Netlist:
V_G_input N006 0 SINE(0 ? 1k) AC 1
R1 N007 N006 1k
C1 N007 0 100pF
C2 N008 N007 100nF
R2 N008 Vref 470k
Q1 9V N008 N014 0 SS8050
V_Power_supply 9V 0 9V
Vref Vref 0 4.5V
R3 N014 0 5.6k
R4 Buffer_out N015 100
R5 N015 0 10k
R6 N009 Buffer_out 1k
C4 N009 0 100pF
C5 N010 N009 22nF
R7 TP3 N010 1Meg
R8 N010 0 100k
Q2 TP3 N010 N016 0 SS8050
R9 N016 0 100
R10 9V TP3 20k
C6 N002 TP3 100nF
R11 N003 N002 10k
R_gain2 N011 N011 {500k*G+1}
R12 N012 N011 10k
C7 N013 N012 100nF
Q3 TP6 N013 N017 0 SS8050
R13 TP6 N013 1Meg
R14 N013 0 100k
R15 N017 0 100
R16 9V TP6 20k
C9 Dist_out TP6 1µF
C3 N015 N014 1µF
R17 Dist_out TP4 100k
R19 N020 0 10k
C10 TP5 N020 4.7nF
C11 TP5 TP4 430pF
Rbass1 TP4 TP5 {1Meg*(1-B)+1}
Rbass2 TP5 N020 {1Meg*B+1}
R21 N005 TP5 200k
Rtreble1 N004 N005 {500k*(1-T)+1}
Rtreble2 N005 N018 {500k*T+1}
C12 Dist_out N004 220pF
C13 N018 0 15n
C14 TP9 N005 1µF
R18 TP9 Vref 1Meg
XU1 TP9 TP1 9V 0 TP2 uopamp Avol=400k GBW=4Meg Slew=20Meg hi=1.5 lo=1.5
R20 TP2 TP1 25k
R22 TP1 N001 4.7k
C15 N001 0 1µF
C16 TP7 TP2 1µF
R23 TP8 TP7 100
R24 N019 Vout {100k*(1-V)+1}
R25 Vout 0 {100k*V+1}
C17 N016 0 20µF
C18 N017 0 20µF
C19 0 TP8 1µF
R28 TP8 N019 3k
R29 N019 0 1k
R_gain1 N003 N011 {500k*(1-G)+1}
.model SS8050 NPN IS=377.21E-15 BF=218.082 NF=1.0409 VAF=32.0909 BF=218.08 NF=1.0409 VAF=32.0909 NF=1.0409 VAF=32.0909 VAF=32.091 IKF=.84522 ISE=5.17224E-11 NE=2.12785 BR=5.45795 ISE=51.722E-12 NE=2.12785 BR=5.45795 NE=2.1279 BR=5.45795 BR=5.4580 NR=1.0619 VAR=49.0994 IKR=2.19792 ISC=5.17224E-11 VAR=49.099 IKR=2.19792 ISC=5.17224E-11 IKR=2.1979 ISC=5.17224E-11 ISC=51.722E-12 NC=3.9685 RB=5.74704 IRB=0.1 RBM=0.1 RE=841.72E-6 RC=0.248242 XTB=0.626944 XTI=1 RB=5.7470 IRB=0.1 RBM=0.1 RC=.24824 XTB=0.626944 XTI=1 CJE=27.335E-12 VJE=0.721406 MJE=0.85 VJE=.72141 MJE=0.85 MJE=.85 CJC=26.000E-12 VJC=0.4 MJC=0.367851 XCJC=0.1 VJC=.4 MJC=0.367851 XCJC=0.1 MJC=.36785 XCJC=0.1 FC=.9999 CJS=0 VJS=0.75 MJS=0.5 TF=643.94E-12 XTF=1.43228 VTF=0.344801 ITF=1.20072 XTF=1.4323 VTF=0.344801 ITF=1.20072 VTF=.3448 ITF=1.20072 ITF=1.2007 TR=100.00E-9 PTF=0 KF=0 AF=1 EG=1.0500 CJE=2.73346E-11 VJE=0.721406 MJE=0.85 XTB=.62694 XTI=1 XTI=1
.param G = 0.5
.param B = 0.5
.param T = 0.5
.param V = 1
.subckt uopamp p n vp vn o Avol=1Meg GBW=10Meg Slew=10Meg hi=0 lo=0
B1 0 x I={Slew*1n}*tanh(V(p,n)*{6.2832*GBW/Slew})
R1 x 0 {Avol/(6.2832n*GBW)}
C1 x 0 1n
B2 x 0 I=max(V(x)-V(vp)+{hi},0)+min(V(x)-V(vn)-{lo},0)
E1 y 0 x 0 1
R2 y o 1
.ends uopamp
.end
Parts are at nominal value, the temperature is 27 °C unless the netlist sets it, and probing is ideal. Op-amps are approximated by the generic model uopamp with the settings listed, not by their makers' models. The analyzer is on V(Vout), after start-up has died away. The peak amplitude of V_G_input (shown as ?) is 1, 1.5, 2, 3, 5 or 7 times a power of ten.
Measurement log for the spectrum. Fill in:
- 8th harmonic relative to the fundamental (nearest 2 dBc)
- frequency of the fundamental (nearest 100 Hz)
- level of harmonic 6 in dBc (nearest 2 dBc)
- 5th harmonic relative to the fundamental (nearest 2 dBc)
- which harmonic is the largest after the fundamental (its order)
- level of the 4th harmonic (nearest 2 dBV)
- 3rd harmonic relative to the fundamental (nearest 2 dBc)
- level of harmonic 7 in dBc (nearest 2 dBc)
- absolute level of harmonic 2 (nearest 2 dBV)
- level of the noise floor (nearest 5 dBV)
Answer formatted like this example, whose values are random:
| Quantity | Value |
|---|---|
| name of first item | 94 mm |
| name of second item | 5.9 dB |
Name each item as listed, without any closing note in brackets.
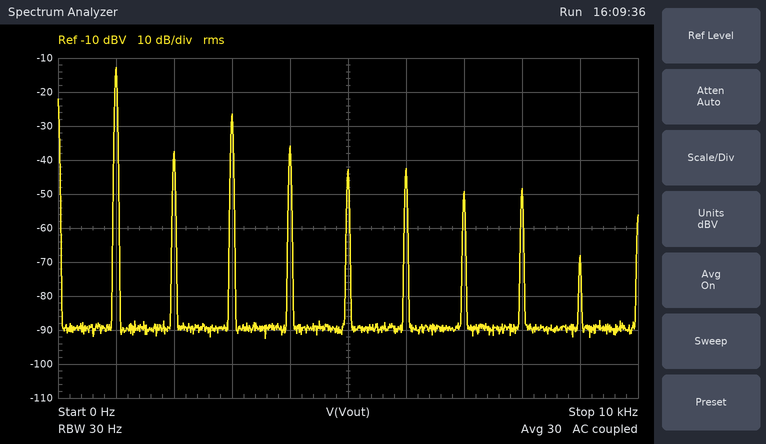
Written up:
| Quantity | Value |
|---|---|
| 8th harmonic relative to the fundamental | -36 dBc |
| frequency of the fundamental | 1.0 kHz |
| level of harmonic 6 in dBc | -30 dBc |
| 5th harmonic relative to the fundamental | -30 dBc |
| which harmonic is the largest after the fundamental | 3 |
| level of the 4th harmonic | -36 dBV |
| 3rd harmonic relative to the fundamental | -14 dBc |
| level of harmonic 7 in dBc | -36 dBc |
| absolute level of harmonic 2 | -38 dBV |
| level of the noise floor | -90 dBV |
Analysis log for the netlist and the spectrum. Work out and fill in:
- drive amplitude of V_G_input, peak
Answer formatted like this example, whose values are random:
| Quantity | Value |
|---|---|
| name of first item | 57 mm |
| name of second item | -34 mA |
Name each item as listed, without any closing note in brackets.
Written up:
| Quantity | Value |
|---|---|
| drive amplitude of V_G_input, peak | 70 mV |
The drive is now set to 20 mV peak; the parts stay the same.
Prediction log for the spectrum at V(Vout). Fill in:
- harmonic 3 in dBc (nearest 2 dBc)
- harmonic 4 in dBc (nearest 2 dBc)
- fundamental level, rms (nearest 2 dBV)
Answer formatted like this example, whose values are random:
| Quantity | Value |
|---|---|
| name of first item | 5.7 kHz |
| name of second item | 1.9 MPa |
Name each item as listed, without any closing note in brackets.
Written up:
| Quantity | Value |
|---|---|
| harmonic 3 in dBc | -26 dBc |
| harmonic 4 in dBc | -36 dBc |
| fundamental level, rms | -18 dBV |
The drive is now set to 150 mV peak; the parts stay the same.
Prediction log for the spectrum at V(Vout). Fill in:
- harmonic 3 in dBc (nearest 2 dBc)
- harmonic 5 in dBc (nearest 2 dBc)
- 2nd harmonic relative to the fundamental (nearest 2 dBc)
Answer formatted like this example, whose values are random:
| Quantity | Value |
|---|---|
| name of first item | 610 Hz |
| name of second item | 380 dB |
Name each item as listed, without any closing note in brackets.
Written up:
| Quantity | Value |
|---|---|
| harmonic 3 in dBc | -18 dBc |
| harmonic 5 in dBc | -28 dBc |
| 2nd harmonic relative to the fundamental | -8 dBc |
